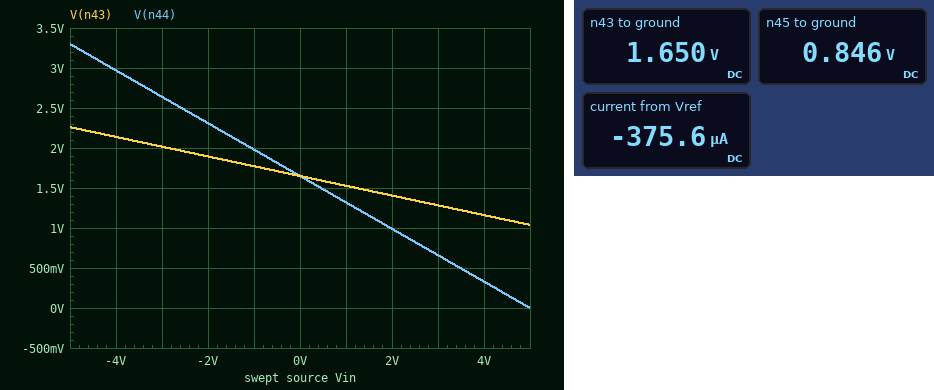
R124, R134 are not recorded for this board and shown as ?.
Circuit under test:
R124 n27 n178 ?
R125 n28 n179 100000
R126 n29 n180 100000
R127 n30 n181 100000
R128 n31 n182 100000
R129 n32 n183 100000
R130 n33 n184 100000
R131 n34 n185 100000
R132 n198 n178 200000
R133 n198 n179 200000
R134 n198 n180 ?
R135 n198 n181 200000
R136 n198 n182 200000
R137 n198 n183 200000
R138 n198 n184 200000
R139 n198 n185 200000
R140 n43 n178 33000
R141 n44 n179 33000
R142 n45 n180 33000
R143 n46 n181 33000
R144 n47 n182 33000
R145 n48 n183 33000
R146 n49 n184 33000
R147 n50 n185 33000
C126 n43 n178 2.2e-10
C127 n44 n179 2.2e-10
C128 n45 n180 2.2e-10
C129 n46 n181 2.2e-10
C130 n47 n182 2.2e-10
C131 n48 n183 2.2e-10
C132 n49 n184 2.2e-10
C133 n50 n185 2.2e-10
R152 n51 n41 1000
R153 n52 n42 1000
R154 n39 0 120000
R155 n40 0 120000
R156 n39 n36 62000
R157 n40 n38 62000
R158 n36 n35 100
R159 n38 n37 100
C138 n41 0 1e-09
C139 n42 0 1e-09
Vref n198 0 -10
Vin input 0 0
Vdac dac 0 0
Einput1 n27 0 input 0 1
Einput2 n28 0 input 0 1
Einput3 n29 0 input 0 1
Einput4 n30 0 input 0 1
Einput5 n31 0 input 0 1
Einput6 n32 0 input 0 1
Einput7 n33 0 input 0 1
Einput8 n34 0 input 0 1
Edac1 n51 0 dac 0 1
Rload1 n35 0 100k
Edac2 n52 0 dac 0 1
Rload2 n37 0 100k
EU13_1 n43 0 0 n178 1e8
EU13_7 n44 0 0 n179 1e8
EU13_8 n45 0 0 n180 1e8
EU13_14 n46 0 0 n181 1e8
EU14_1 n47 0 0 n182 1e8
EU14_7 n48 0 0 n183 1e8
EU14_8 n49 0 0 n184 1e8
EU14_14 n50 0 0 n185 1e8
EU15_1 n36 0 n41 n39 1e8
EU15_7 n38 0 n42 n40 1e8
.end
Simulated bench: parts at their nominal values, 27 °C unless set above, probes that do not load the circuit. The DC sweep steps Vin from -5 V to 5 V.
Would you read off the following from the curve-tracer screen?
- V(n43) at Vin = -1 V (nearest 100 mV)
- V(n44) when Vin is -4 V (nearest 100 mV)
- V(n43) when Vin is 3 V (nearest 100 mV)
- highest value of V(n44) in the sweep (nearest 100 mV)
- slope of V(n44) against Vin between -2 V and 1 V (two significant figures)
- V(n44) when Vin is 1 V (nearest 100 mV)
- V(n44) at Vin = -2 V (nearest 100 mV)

1.8 V
3.0 V
1.3 V
3.3 V
-0.33 V/V
1.3 V
2.3 V
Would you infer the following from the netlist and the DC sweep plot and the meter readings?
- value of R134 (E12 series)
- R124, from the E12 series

390 kΩ
270 kΩ
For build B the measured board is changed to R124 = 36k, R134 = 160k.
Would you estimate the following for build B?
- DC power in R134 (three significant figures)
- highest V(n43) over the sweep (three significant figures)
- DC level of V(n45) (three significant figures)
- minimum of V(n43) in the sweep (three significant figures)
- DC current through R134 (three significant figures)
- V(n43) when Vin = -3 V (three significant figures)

625 µW
6.23 V
2.06 V
-2.93 V
62.5 µA
4.40 V
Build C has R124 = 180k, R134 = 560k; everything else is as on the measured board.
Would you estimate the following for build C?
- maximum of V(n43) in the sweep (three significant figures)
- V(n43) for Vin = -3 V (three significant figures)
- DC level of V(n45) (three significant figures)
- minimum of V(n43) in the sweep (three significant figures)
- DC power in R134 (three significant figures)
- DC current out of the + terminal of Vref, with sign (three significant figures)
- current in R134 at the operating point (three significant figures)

2.57 V
2.20 V
589 mV
733 mV
179 µW
-368 µA
17.9 µA
